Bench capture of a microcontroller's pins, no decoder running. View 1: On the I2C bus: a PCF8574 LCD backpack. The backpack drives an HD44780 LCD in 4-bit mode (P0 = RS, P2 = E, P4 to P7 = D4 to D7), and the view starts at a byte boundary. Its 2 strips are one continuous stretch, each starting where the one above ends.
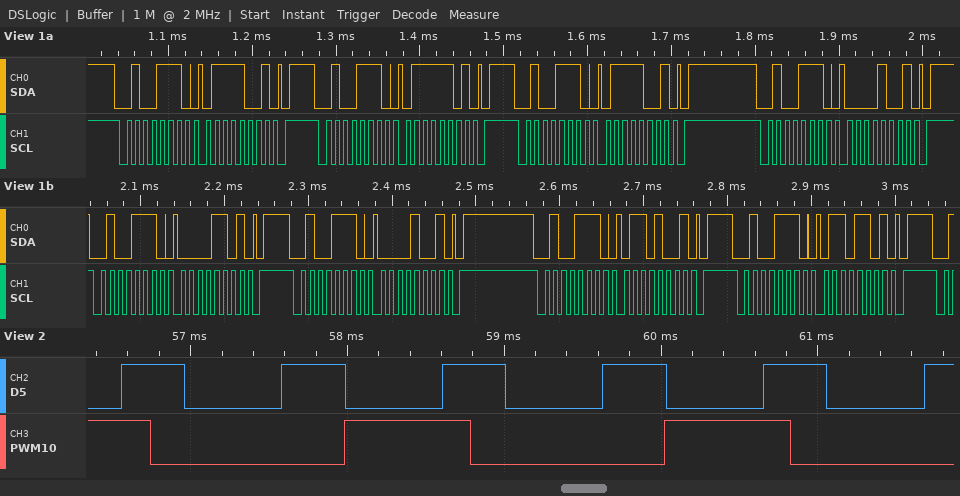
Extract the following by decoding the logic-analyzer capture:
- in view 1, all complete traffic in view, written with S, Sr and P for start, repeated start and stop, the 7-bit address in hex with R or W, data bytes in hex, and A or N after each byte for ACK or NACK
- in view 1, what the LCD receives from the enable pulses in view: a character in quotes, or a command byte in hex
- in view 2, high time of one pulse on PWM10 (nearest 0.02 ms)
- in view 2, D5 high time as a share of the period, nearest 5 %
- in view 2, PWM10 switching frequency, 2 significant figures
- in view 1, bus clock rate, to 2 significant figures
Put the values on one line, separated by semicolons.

S 27W A 79 A P S 27W A 7D A P S 27W A 79 A P S 27W A 09 A P S 27W A 0D A P S 27W A 09 A P S 27W A 69 A P S 27W A 6D A P; 'p'; 0.80 ms; 40 %; 490 Hz; 100 kHz
